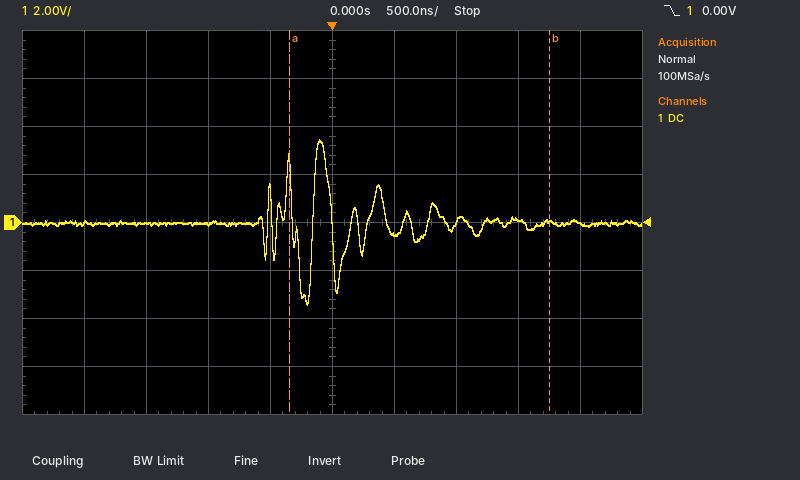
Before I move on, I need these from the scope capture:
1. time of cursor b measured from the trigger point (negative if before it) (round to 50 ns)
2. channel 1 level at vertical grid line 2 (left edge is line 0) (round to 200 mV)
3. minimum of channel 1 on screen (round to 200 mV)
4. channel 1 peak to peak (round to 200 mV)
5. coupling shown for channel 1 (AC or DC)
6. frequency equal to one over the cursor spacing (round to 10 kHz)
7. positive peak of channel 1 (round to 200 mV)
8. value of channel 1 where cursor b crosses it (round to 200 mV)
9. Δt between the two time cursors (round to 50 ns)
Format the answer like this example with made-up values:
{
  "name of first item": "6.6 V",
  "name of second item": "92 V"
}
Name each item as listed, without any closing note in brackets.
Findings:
{
  "time of cursor b measured from the trigger point (negative if before it)": "+1.75 µs",
  "channel 1 level at vertical grid line 2 (left edge is line 0)": "0.0 V",
  "minimum of channel 1 on screen": "-3.4 V",
  "channel 1 peak to peak": "6.8 V",
  "coupling shown for channel 1": "DC",
  "frequency equal to one over the cursor spacing": "480 kHz",
  "positive peak of channel 1": "3.4 V",
  "value of channel 1 where cursor b crosses it": "0.0 V",
  "Δt between the two time cursors": "2.10 µs"
}
